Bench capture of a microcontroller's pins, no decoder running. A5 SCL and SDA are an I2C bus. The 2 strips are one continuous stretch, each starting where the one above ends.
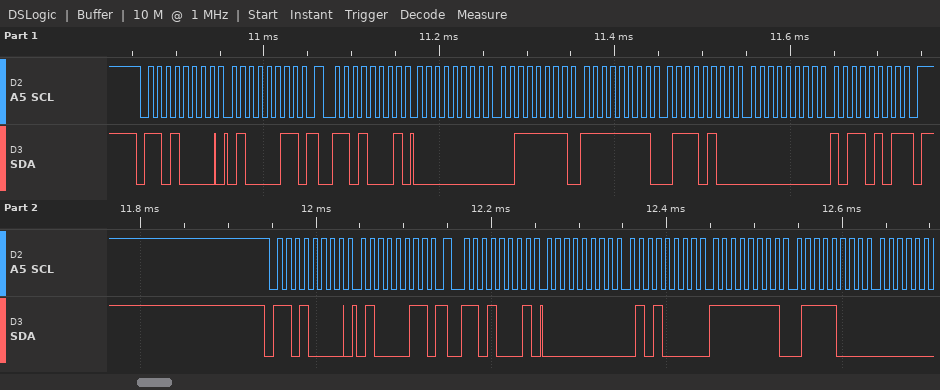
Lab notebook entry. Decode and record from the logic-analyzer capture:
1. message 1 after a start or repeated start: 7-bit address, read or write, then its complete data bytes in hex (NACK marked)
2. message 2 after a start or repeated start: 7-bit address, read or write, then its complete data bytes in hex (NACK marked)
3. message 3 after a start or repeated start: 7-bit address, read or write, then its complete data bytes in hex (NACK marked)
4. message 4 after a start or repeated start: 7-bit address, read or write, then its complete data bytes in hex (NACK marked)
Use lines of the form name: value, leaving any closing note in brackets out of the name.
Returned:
message 1 after a start or repeated start: 7-bit address, read or write, then its complete data bytes in hex: 0x68 write: 43
message 2 after a start or repeated start: 7-bit address, read or write, then its complete data bytes in hex: 0x68 read: 00 3F FF 74 00 B5 NACK
message 3 after a start or repeated start: 7-bit address, read or write, then its complete data bytes in hex: 0x68 write: 43
message 4 after a start or repeated start: 7-bit address, read or write, then its complete data bytes in hex: 0x68 read: 00 50 FF 78
